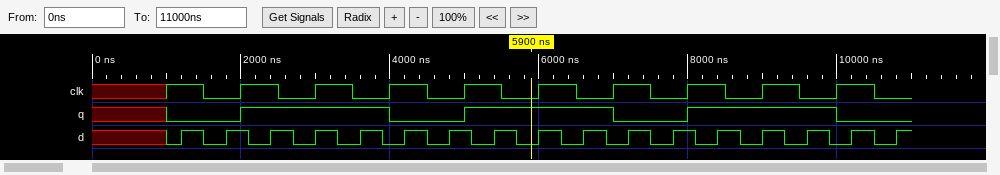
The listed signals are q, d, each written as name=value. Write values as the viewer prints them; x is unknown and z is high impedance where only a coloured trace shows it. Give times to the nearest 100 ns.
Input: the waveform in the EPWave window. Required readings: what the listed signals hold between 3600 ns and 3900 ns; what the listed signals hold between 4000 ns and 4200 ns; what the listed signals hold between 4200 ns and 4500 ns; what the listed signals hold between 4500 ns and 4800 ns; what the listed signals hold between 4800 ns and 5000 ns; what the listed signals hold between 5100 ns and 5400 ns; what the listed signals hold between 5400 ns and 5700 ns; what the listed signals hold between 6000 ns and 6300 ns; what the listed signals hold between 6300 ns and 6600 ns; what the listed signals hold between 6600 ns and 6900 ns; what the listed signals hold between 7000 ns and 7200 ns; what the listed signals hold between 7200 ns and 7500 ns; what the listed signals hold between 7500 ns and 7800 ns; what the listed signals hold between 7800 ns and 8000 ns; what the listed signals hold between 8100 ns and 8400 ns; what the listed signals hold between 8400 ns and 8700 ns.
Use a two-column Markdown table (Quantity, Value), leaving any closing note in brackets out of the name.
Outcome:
| Quantity | Value |
|---|---|
| what the listed signals hold between 3600 ns and 3900 ns | q=1, d=1 |
| what the listed signals hold between 4000 ns and 4200 ns | q=0, d=0 |
| what the listed signals hold between 4200 ns and 4500 ns | q=0, d=1 |
| what the listed signals hold between 4500 ns and 4800 ns | q=0, d=0 |
| what the listed signals hold between 4800 ns and 5000 ns | q=0, d=1 |
| what the listed signals hold between 5100 ns and 5400 ns | q=1, d=0 |
| what the listed signals hold between 5400 ns and 5700 ns | q=1, d=1 |
| what the listed signals hold between 6000 ns and 6300 ns | q=1, d=1 |
| what the listed signals hold between 6300 ns and 6600 ns | q=1, d=0 |
| what the listed signals hold between 6600 ns and 6900 ns | q=1, d=1 |
| what the listed signals hold between 7000 ns and 7200 ns | q=0, d=0 |
| what the listed signals hold between 7200 ns and 7500 ns | q=0, d=1 |
| what the listed signals hold between 7500 ns and 7800 ns | q=0, d=0 |
| what the listed signals hold between 7800 ns and 8000 ns | q=0, d=1 |
| what the listed signals hold between 8100 ns and 8400 ns | q=1, d=0 |
| what the listed signals hold between 8400 ns and 8700 ns | q=1, d=1 |
